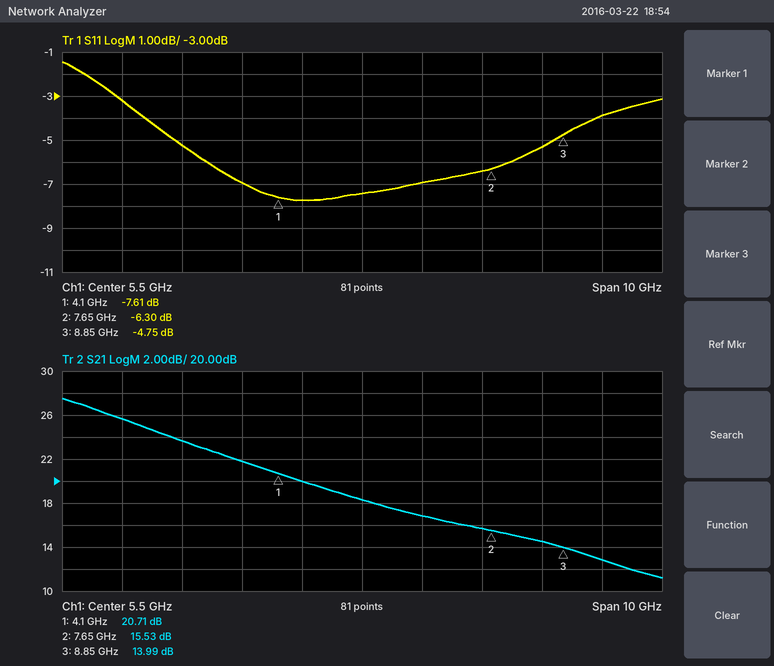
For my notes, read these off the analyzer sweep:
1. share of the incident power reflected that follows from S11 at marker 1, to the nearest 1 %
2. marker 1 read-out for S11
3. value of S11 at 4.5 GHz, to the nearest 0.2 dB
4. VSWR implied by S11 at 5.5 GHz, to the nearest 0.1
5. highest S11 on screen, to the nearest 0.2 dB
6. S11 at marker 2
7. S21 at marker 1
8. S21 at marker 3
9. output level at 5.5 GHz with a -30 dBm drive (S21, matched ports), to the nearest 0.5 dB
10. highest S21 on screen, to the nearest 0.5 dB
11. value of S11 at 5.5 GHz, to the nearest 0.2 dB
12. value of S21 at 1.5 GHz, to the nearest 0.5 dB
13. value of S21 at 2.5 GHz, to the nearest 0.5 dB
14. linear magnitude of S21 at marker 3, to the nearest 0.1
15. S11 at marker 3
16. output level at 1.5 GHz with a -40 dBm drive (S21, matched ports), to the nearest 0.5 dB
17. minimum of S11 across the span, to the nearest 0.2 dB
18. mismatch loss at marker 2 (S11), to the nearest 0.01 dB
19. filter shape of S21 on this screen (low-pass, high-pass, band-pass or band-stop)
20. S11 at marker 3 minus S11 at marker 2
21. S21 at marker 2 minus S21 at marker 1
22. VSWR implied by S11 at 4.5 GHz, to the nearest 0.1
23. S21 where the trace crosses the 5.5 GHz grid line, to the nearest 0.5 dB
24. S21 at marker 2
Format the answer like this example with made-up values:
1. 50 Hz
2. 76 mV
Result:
1. 17 %
2. -7.61 dB
3. -7.8 dB
4. 2.5
5. -1.4 dB
6. -6.30 dB
7. 20.71 dB
8. 13.99 dB
9. -11.5 dBm
10. 27.5 dB
11. -7.4 dB
12. 25.5 dB
13. 23.5 dB
14. 5.0
15. -4.75 dB
16. -14.5 dBm
17. -7.8 dB
18. 1.16 dB
19. low-pass
20. 1.55 dB
21. -5.18 dB
22. 2.4
23. 18.5 dB
24. 15.53 dB
